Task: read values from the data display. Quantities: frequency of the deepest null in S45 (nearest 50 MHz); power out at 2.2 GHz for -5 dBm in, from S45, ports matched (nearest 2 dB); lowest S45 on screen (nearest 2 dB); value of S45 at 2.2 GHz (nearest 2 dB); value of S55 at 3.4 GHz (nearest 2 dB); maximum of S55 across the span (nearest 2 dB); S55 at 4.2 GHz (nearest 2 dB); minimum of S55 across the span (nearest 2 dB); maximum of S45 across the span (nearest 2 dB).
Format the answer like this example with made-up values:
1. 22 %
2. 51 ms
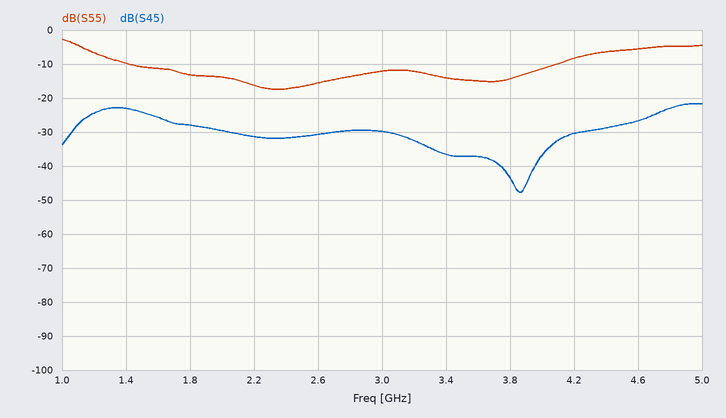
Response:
1. 3.85 GHz
2. -36 dBm
3. -48 dB
4. -32 dB
5. -14 dB
6. -2 dB
7. -8 dB
8. -18 dB
9. -22 dB
